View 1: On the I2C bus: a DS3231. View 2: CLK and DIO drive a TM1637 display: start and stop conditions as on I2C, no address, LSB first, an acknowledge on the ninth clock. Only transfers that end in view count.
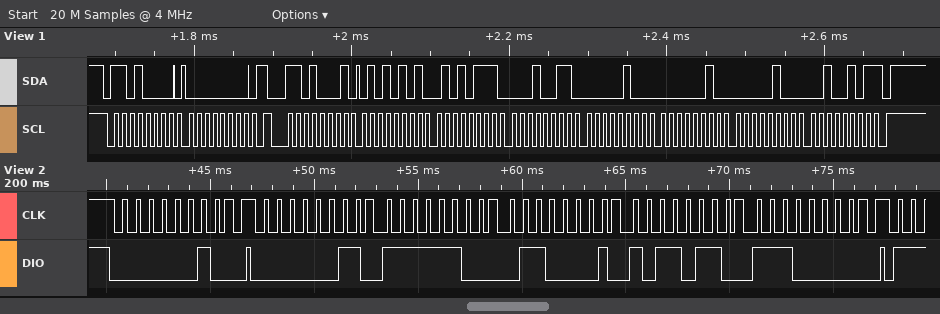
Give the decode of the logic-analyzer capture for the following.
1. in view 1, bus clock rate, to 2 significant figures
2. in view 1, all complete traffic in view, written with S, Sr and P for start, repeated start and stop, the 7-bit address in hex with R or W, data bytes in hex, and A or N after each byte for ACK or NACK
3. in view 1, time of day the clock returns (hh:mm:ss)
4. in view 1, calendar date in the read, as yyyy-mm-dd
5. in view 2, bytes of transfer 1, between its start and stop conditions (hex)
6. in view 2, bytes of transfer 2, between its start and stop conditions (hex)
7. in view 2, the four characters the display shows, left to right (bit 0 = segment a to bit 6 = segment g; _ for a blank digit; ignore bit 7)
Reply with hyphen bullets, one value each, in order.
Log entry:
- 100 kHz
- S 68W A 00 A Sr 68R A 55 A 57 A 13 A 04 A 02 A 04 A 25 N P
- 13:57:55
- 2025-04-02
- 40
- C0 3F 86 6D 07
- 0157
